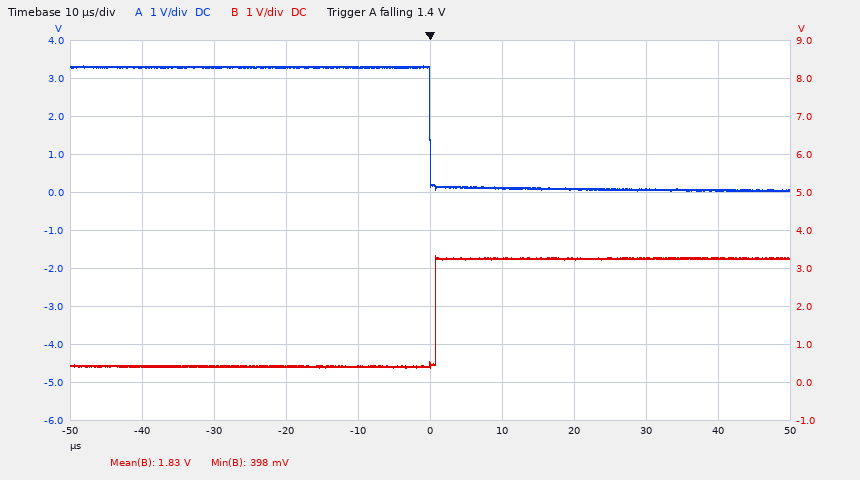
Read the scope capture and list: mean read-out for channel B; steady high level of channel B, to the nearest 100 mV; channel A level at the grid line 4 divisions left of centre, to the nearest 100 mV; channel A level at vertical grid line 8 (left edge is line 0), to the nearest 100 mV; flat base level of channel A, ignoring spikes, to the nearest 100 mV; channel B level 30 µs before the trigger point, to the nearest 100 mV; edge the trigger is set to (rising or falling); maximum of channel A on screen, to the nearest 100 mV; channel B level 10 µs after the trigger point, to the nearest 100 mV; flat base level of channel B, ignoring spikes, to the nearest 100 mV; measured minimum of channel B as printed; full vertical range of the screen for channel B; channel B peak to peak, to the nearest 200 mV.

1.83 V
3.3 V
3.3 V
100 mV
100 mV
400 mV
falling
3.3 V
3.3 V
400 mV
398 mV
10 V
3.0 V
